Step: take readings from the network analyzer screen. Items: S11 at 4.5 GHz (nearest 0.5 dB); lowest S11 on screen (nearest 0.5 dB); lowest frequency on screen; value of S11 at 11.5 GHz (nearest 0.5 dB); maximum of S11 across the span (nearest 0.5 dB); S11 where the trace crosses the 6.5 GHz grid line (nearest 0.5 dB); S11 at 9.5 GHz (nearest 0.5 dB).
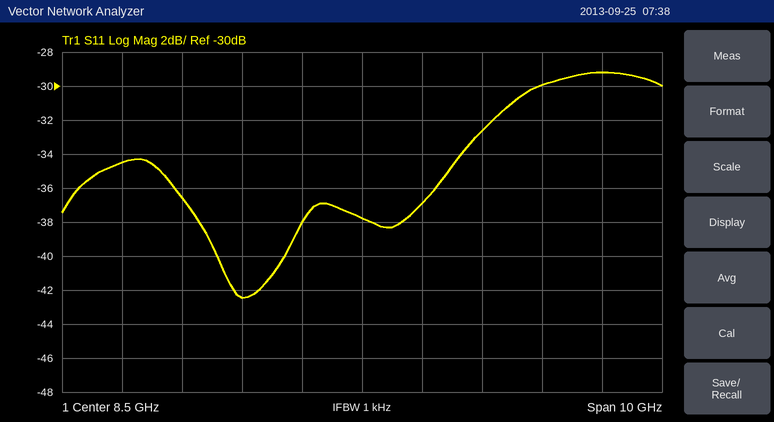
-34.5 dB
-42.5 dB
3.5 GHz
-30.0 dB
-29.0 dB
-42.5 dB
-37.0 dB
